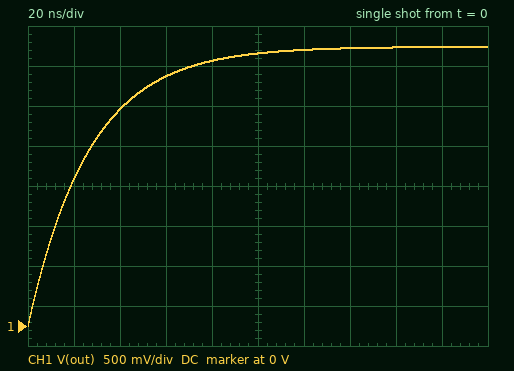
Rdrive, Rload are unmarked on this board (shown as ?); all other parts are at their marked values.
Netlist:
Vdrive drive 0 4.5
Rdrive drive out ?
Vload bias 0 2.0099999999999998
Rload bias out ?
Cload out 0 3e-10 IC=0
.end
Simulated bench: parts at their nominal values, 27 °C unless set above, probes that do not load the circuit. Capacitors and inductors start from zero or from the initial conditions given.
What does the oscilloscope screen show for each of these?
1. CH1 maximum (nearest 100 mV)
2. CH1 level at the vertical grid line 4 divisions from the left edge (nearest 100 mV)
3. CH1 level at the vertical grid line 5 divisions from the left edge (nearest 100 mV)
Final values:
3.5 V
3.3 V
3.4 V
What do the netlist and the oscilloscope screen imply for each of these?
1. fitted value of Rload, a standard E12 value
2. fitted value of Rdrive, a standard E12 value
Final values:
220 Ω
150 Ω
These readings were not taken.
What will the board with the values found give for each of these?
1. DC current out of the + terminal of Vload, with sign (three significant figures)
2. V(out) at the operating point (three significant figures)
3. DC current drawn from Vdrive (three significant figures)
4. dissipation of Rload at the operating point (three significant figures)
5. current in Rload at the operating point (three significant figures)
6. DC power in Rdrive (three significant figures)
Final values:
-6.73 mA
3.49 V
6.73 mA
9.96 mW
6.73 mA
6.79 mW
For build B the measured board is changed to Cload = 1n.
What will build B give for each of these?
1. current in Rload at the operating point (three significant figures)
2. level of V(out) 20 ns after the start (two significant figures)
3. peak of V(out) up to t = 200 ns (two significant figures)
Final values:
6.73 mA
700 mV
3.1 V
